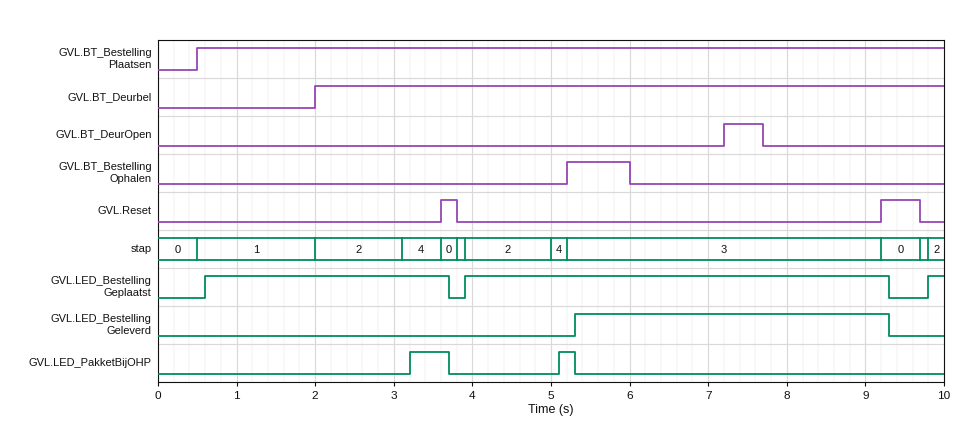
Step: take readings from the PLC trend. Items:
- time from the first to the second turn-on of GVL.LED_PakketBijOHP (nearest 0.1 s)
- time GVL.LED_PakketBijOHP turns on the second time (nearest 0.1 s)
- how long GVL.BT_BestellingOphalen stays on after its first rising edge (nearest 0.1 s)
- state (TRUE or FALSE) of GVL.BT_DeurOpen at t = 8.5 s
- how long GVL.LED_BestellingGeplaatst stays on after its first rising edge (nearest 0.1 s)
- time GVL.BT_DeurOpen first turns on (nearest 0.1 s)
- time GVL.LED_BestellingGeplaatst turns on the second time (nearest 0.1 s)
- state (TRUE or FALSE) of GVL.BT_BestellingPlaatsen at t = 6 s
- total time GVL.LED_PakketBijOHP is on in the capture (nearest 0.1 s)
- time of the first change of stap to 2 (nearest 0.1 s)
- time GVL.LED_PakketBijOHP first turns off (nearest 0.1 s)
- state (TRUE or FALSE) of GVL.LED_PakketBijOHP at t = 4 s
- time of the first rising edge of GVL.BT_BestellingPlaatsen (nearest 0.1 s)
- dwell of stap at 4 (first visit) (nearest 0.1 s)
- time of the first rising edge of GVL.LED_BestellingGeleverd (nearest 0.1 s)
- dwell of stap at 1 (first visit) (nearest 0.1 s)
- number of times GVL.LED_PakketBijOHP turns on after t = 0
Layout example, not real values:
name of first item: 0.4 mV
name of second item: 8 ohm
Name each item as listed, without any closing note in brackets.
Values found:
time from the first to the second turn-on of GVL.LED_PakketBijOHP: 1.9 s
time GVL.LED_PakketBijOHP turns on the second time: 5.1 s
how long GVL.BT_BestellingOphalen stays on after its first rising edge: 0.8 s
state (TRUE or FALSE) of GVL.BT_DeurOpen at t = 8.5 s: FALSE
how long GVL.LED_BestellingGeplaatst stays on after its first rising edge: 3.1 s
time GVL.BT_DeurOpen first turns on: 7.2 s
time GVL.LED_BestellingGeplaatst turns on the second time: 3.9 s
state (TRUE or FALSE) of GVL.BT_BestellingPlaatsen at t = 6 s: TRUE
total time GVL.LED_PakketBijOHP is on in the capture: 0.7 s
time of the first change of stap to 2: 2.0 s
time GVL.LED_PakketBijOHP first turns off: 3.7 s
state (TRUE or FALSE) of GVL.LED_PakketBijOHP at t = 4 s: FALSE
time of the first rising edge of GVL.BT_BestellingPlaatsen: 0.5 s
dwell of stap at 4 (first visit): 0.5 s
time of the first rising edge of GVL.LED_BestellingGeleverd: 5.3 s
dwell of stap at 1 (first visit): 1.5 s
number of times GVL.LED_PakketBijOHP turns on after t = 0: 2
